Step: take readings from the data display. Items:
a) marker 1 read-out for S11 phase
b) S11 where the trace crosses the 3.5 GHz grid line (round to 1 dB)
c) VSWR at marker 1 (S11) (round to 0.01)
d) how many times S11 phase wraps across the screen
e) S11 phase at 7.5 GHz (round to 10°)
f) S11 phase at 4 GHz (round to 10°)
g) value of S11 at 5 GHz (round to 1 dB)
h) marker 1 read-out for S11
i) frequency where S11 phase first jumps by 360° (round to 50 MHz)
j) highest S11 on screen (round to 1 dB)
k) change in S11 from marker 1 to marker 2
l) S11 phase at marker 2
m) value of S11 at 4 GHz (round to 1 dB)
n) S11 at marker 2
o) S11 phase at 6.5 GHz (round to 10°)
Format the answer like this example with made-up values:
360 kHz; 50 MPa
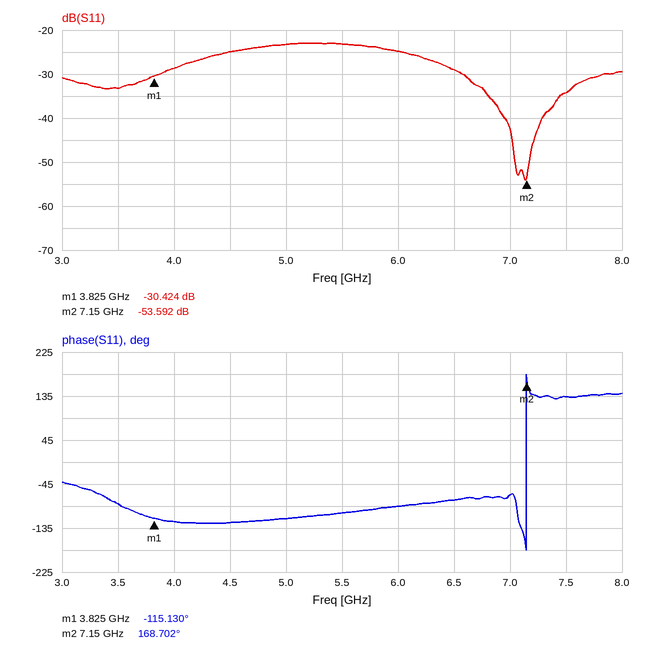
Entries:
-115.130°; -33 dB; 1.06; 1; 130°; -120°; -23 dB; -30.424 dB; 7.15 GHz; -23 dB; -23.168 dB; 168.702°; -29 dB; -53.592 dB; -80°
